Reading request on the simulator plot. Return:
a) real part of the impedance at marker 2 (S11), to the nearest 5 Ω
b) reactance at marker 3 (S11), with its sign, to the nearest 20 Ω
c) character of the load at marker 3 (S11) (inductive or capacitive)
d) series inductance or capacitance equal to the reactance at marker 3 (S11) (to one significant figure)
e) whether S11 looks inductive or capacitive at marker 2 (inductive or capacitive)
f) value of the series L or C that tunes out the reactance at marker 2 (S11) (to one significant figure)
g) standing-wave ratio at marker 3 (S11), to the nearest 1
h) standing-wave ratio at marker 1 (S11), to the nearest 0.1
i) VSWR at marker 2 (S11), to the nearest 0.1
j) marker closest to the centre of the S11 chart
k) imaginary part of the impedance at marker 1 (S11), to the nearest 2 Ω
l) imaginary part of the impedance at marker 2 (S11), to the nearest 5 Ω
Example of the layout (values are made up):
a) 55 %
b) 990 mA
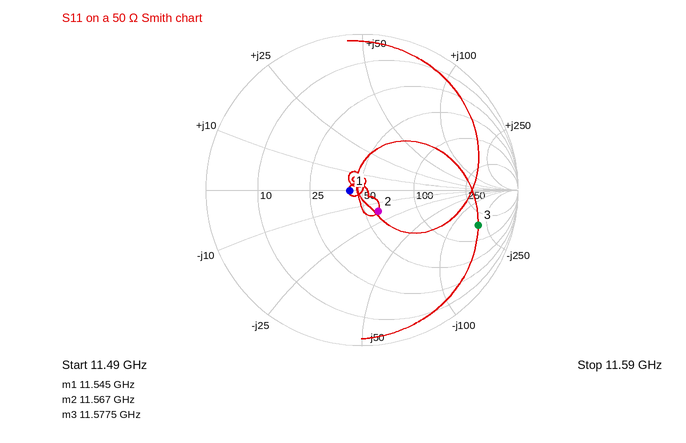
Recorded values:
a) 60 Ω
b) -200 Ω
c) capacitive
d) 70 fF
e) capacitive
f) 200 pH
g) 8
h) 1.2
i) 1.4
j) marker 1
k) 0 Ω
l) -15 Ω
